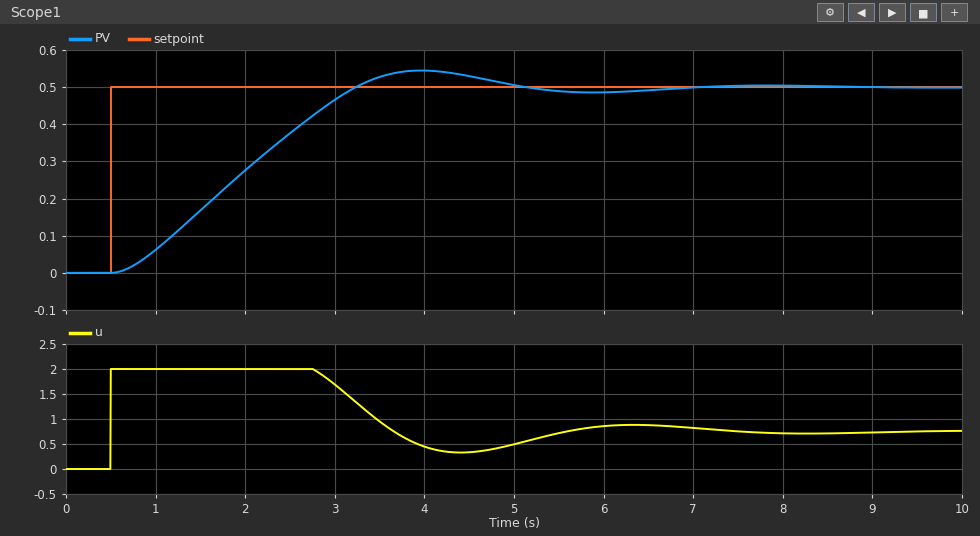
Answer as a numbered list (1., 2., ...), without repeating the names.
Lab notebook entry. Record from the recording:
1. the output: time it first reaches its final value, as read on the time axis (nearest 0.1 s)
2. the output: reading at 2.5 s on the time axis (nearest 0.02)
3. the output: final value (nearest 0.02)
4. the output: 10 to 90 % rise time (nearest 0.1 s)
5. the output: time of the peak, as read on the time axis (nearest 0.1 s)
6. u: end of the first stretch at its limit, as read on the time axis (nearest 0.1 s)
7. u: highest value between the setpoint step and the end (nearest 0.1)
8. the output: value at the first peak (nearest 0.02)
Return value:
1. 3.2 s
2. 0.38
3. 0.50
4. 2.0 s
5. 4.0 s
6. 2.8 s
7. 2.0
8. 0.54
